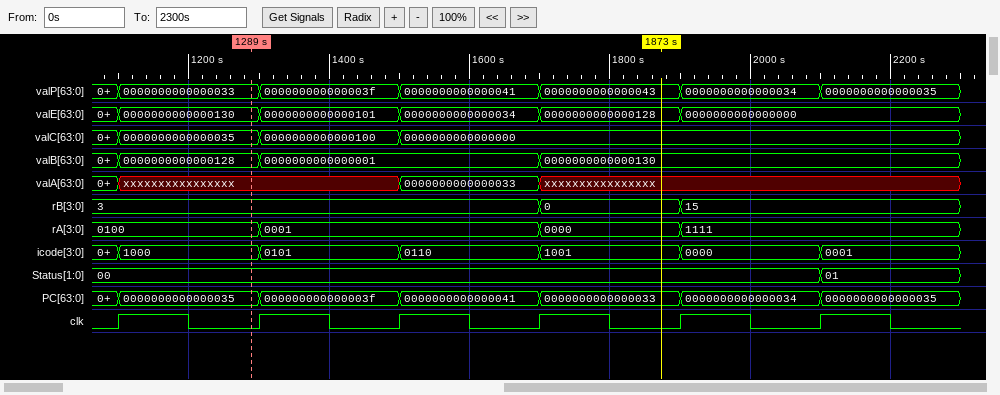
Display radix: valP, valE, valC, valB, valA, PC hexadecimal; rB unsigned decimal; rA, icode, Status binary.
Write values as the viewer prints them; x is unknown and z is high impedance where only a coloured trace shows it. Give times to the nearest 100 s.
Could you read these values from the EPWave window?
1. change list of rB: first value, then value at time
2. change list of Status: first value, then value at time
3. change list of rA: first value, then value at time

3, 0 at 1700 s, 15 at 1900 s
00, 01 at 2100 s
0100, 0001 at 1300 s, 0000 at 1700 s, 1111 at 1900 s
